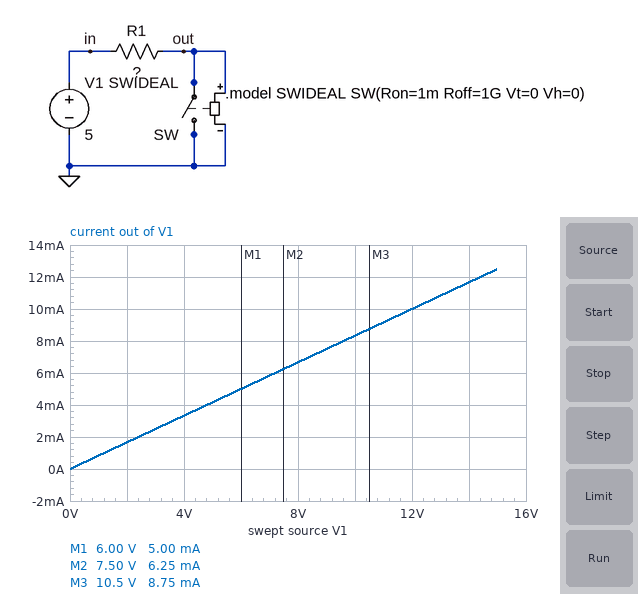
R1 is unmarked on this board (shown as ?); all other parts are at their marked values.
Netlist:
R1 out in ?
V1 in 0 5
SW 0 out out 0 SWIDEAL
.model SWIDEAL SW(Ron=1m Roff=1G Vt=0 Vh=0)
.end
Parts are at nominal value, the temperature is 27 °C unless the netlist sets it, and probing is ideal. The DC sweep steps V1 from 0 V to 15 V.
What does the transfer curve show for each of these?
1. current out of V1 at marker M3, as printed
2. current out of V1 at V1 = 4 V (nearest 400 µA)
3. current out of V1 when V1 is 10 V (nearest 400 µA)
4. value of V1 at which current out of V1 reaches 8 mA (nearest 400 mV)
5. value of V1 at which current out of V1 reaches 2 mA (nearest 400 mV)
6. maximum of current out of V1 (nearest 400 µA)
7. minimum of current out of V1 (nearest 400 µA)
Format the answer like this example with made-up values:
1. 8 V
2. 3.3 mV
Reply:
1. 8.75 mA
2. 3.2 mA
3. 8.4 mA
4. 9.6 V
5. 2.4 V
6. 12.4 mA
7. 0 A
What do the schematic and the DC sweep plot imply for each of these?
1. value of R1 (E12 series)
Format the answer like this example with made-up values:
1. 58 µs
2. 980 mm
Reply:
1. 1.2 kΩ
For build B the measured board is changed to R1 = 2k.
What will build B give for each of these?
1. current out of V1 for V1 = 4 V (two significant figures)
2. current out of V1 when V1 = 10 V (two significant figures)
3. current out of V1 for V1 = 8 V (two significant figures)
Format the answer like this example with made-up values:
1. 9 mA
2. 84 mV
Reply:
1. 2.0 mA
2. 5.0 mA
3. 4.0 mA
